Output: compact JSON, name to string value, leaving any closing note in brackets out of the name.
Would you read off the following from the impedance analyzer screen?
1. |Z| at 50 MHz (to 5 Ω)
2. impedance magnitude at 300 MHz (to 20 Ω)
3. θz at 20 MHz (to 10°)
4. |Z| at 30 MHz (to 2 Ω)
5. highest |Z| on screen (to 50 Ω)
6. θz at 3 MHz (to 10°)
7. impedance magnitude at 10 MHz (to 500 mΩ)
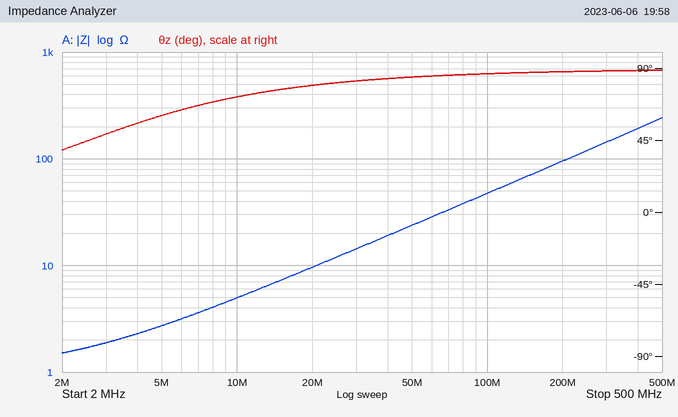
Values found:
{"|Z| at 50 MHz": "25 Ω", "impedance magnitude at 300 MHz": "140 Ω", "θz at 20 MHz": "80°", "|Z| at 30 MHz": "14 Ω", "highest |Z| on screen": "250 Ω", "θz at 3 MHz": "50°", "impedance magnitude at 10 MHz": "5.0 Ω"}
